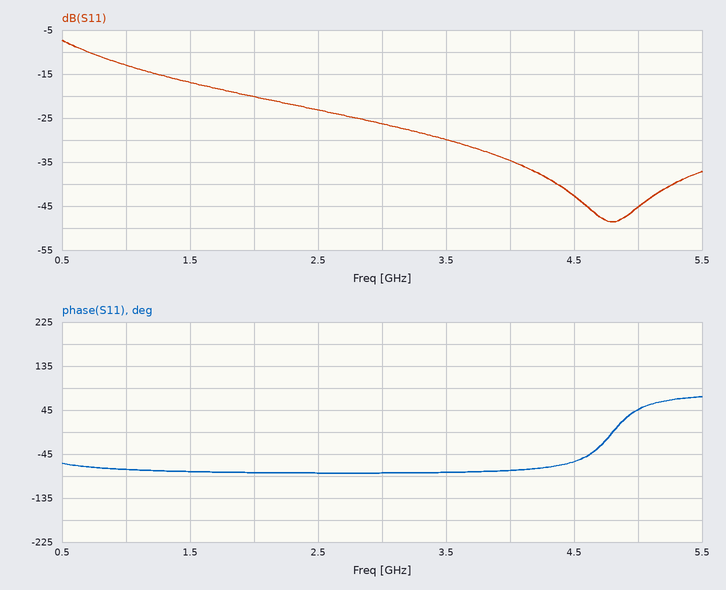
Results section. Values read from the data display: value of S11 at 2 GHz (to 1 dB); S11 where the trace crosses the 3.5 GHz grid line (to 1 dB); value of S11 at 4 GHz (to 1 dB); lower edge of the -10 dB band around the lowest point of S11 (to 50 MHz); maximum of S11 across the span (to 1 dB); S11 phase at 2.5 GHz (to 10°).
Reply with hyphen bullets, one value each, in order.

- -20 dB
- -30 dB
- -35 dB
- 700 MHz
- -7 dB
- -80°
